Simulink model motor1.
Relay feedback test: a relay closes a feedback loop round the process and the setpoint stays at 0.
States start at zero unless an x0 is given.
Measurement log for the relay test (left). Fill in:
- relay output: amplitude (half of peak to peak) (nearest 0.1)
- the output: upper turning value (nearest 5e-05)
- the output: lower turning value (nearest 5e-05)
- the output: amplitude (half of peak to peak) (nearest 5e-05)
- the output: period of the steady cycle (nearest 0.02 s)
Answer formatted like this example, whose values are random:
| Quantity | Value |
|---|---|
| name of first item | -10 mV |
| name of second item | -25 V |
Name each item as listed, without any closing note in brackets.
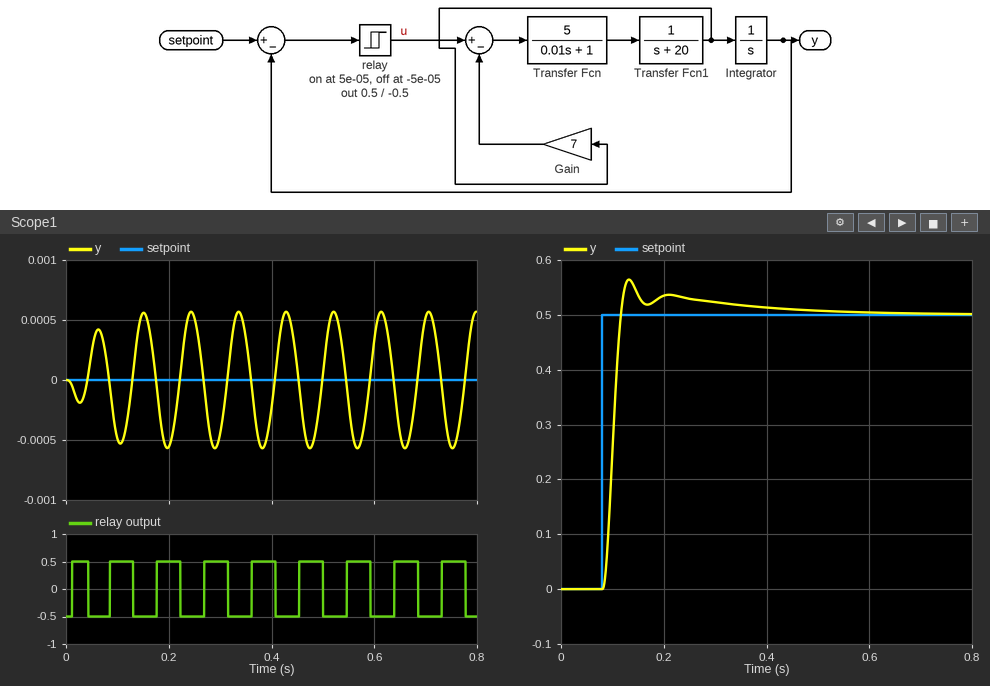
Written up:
| Quantity | Value |
|---|---|
| relay output: amplitude (half of peak to peak) | 0.5 |
| the output: upper turning value | 0.00055 |
| the output: lower turning value | -0.00055 |
| the output: amplitude (half of peak to peak) | 0.00055 |
| the output: period of the steady cycle | 0.10 s |
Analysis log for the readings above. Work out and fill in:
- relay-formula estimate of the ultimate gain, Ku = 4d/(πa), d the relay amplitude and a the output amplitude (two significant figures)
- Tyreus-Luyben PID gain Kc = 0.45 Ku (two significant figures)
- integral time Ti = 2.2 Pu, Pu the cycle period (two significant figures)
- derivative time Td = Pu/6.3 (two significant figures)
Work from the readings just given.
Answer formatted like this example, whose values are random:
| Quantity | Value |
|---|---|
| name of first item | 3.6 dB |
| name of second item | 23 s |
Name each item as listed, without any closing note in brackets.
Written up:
| Quantity | Value |
|---|---|
| relay-formula estimate of the ultimate gain, Ku = 4d/(πa), d the relay amplitude and a the output amplitude | 1200 |
| Tyreus-Luyben PID gain Kc = 0.45 Ku | 540 |
| integral time Ti = 2.2 Pu, Pu the cycle period | 0.22 s |
| derivative time Td = Pu/6.3 | 0.016 s |
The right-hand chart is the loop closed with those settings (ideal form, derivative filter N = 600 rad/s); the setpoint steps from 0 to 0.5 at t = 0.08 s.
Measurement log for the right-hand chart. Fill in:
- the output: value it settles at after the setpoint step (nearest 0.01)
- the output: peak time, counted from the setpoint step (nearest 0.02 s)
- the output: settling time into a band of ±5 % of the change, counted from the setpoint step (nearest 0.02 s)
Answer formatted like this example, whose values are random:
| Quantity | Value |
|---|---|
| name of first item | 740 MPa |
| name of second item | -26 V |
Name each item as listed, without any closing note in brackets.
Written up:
| Quantity | Value |
|---|---|
| the output: value it settles at after the setpoint step | 0.50 |
| the output: peak time, counted from the setpoint step | 0.06 s |
| the output: settling time into a band of ±5 % of the change, counted from the setpoint step | 0.20 s |
